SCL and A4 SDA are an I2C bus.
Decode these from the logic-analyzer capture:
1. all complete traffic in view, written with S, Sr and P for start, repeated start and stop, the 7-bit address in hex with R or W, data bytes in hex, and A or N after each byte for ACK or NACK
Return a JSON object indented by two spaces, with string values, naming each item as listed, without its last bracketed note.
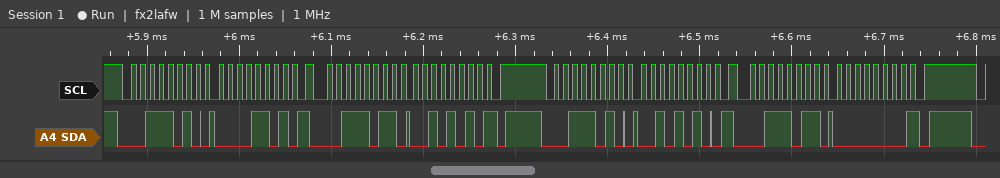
{
  "all complete traffic in view, written with S, Sr and P for start, repeated start and stop, the 7-bit address in hex with R or W, data bytes in hex, and A or N after each byte for ACK or NACK": "S 1DW A 0D A Sr 1DR A 2A N P S 1DW A 2A A Sr 1DR A 00 N P"
}
